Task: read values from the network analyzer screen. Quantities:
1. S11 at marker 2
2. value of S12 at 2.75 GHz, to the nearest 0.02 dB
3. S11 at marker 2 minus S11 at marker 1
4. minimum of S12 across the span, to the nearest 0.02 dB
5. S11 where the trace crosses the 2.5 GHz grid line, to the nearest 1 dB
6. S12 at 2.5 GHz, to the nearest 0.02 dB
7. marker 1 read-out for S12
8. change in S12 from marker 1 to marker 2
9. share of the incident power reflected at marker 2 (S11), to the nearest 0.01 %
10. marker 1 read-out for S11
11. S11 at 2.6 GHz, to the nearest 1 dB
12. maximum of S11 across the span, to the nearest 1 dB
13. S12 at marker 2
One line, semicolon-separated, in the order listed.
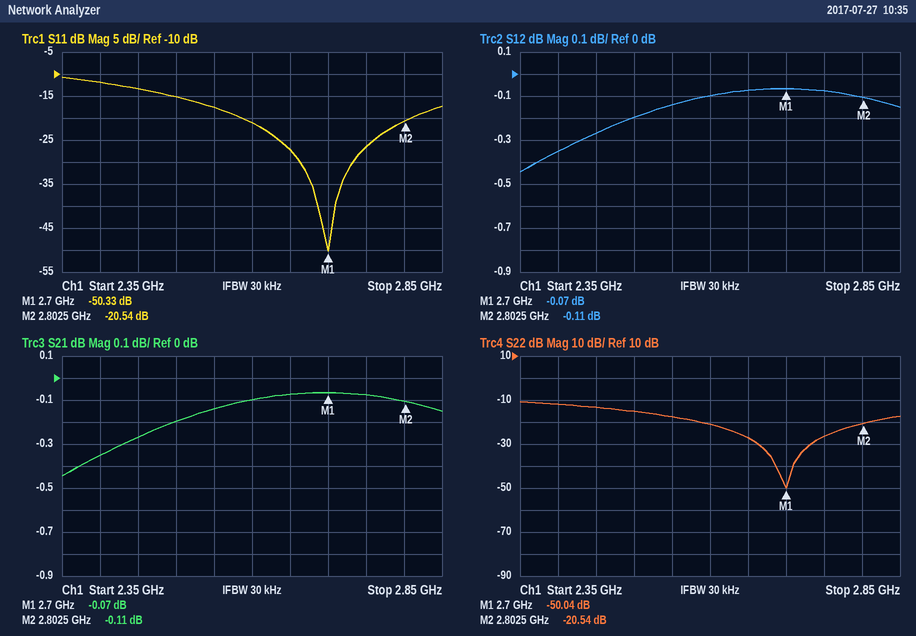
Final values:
-20.54 dB; -0.08 dB; 29.79 dB; -0.44 dB; -15 dB; -0.20 dB; -0.07 dB; -0.04 dB; 0.88 %; -50.33 dB; -21 dB; -11 dB; -0.11 dB
